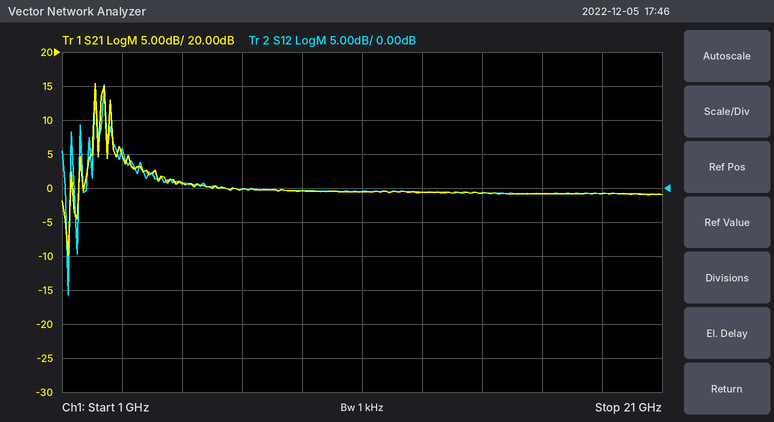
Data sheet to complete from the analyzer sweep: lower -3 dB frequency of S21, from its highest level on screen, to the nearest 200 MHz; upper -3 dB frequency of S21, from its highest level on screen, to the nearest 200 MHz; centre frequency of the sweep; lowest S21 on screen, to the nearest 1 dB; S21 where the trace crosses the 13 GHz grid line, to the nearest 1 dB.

2.0 GHz
2.2 GHz
11 GHz
-10 dB
-1 dB
